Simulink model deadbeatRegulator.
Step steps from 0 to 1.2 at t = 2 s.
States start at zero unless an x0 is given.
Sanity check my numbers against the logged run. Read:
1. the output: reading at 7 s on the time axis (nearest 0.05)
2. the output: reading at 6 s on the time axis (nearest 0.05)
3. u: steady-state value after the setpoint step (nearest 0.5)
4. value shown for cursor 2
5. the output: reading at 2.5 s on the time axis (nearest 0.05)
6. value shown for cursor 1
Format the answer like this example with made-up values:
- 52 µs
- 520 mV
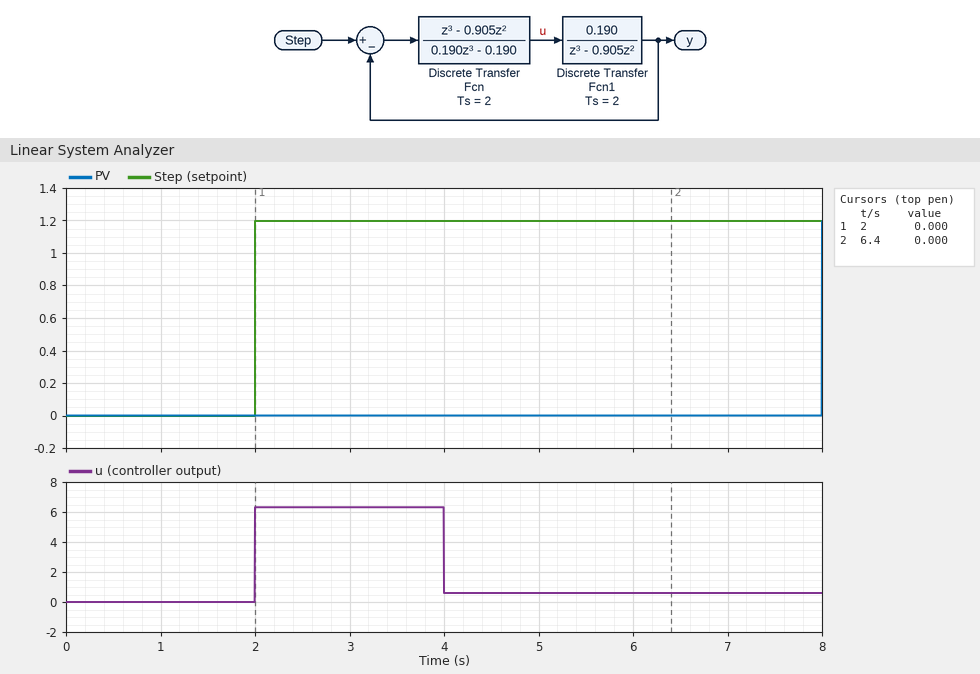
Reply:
- 0.00
- 0.00
- 0.5
- 0.000
- 0.00
- 0.000
